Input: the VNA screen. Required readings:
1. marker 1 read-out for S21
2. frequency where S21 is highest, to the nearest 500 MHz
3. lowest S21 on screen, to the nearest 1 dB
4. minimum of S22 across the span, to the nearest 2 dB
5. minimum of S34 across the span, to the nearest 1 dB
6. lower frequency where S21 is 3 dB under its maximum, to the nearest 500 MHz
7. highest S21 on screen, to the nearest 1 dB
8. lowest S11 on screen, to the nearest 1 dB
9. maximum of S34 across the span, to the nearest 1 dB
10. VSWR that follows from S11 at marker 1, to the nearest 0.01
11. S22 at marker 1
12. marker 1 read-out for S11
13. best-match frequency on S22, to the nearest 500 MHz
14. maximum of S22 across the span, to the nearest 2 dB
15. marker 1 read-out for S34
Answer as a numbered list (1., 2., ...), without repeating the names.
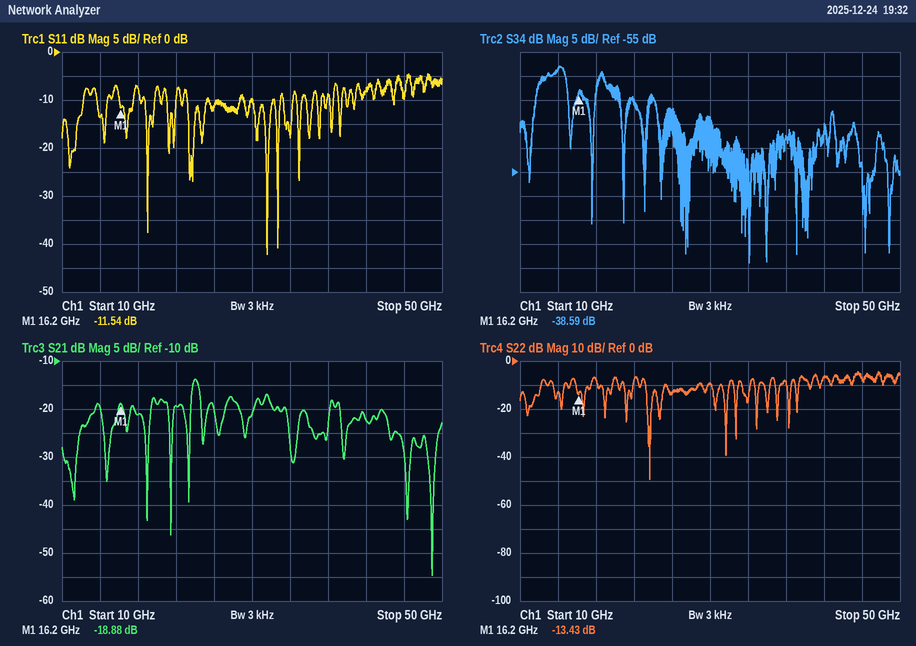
1. -18.88 dB
2. 24.0 GHz
3. -55 dB
4. -50 dB
5. -74 dB
6. 23.5 GHz
7. -14 dB
8. -42 dB
9. -33 dB
10. 1.72
11. -13.43 dB
12. -11.54 dB
13. 23.5 GHz
14. -4 dB
15. -38.59 dB
